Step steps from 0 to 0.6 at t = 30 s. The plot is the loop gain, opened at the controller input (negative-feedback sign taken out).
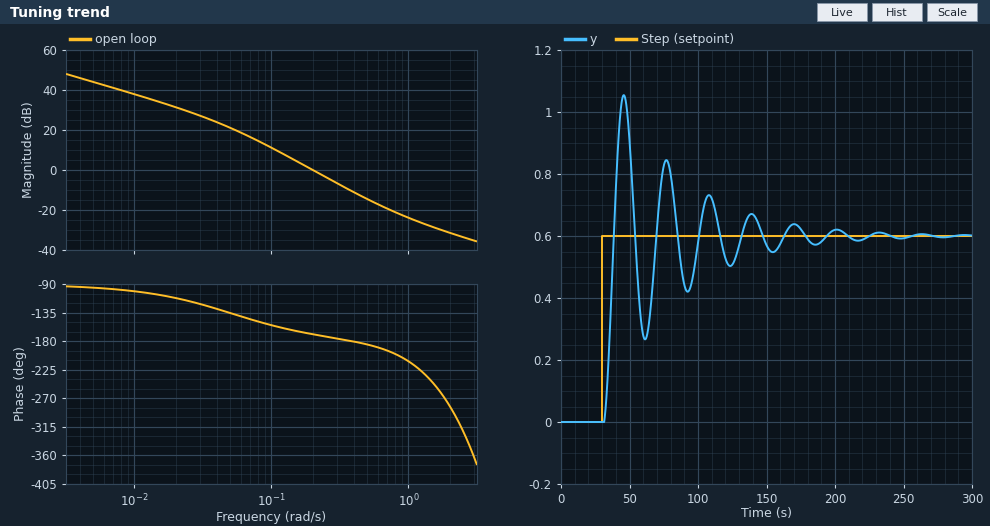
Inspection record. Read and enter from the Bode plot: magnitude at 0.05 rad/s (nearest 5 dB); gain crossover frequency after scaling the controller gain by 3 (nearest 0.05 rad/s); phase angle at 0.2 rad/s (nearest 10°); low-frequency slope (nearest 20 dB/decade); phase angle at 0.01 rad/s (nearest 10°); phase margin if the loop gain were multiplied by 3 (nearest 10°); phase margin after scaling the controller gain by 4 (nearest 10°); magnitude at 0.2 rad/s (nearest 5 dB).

20 dB
0.35 rad/s
-170°
-20 dB/decade
-100°
0°
0°
0 dB
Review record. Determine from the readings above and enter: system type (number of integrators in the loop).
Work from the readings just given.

1
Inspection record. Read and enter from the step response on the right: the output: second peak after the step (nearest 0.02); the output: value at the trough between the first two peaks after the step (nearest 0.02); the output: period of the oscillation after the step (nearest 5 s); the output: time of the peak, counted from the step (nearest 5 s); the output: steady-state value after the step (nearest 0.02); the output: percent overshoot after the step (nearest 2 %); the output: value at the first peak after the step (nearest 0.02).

0.84
0.26
30 s
15 s
0.60
76 %
1.06
